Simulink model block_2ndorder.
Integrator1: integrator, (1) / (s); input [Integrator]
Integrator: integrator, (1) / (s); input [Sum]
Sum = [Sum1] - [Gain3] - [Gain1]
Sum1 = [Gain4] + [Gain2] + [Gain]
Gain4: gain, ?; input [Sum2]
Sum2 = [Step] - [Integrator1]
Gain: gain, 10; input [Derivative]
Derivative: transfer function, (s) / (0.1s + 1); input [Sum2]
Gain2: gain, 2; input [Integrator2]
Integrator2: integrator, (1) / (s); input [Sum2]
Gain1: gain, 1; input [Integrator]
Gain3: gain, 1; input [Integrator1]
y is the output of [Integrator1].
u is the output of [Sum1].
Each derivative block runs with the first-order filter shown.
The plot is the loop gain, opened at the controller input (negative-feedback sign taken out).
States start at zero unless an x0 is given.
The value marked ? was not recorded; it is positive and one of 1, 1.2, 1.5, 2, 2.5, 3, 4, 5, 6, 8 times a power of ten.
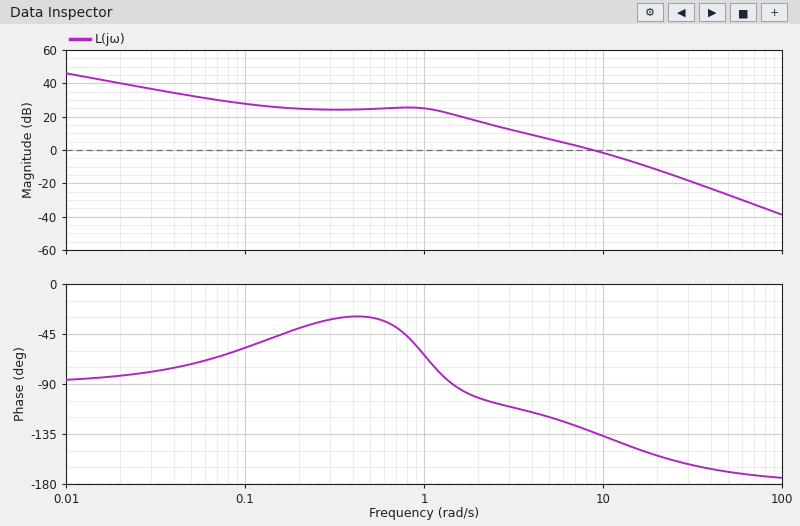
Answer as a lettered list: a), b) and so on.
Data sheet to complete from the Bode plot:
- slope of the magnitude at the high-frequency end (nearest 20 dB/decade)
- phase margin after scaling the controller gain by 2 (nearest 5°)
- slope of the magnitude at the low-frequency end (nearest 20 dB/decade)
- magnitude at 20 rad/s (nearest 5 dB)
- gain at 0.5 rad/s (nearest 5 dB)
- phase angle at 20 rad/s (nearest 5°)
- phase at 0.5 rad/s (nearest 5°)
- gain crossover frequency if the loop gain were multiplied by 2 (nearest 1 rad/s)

a) -40 dB/decade
b) 35°
c) -20 dB/decade
d) -10 dB
e) 25 dB
f) -155°
g) -30°
h) 14 rad/s
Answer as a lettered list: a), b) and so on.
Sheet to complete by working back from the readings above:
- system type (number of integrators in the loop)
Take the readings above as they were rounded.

a) 1
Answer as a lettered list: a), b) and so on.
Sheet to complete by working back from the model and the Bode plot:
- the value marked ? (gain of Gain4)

a) 15
